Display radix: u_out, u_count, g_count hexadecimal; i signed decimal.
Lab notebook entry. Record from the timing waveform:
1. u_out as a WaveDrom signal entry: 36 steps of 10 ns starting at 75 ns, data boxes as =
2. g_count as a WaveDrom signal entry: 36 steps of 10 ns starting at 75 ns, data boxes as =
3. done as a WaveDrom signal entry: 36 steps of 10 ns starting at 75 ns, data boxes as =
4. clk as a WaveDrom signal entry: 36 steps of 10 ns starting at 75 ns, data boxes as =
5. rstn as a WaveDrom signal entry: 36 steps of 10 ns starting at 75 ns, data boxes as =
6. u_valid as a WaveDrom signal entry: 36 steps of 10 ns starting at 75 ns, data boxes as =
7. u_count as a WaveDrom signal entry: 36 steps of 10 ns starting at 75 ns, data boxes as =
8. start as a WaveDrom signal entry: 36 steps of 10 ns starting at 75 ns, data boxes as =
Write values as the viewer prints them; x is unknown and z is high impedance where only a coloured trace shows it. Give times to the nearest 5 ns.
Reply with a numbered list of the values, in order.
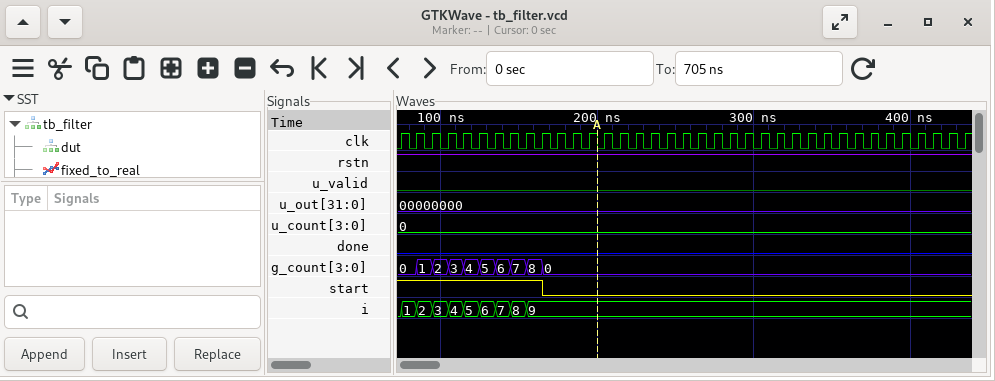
1. {name: 'u_out', wave: '=...................................', data: '00000000'}
2. {name: 'g_count', wave: '==========..........................', data: '0 1 2 3 4 5 6 7 8 0'}
3. {name: 'done', wave: '0...................................'}
4. {name: 'clk', wave: 'p...................................'}
5. {name: 'rstn', wave: '1...................................'}
6. {name: 'u_valid', wave: '0...................................'}
7. {name: 'u_count', wave: '=...................................', data: '0'}
8. {name: 'start', wave: '1........0..........................'}
